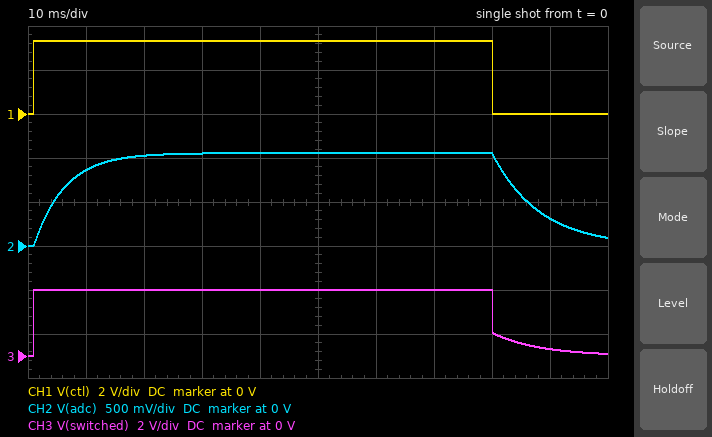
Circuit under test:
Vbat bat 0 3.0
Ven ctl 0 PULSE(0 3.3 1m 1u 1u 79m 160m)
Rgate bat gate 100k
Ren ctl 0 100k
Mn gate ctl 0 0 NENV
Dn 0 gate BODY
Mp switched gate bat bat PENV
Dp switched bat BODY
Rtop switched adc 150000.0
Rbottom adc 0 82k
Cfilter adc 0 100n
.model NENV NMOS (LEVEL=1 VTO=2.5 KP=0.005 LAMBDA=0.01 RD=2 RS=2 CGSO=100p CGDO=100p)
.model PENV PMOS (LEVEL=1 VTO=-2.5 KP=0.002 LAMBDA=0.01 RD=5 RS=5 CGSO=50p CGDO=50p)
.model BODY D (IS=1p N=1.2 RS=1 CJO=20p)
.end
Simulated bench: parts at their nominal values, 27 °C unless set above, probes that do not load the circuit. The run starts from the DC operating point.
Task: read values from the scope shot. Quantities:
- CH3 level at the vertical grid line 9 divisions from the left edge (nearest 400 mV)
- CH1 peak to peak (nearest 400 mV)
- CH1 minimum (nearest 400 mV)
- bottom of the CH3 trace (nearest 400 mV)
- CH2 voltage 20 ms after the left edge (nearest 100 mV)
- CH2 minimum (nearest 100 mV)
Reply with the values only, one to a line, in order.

400 mV
3.2 V
0 V
0 V
1.0 V
0 V
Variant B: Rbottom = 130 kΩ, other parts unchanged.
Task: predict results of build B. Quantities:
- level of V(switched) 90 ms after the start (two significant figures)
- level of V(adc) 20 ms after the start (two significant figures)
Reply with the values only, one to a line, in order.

640 mV
1.3 V
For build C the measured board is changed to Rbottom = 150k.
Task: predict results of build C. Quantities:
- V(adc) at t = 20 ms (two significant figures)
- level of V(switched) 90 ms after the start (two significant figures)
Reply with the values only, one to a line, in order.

1.4 V
770 mV
